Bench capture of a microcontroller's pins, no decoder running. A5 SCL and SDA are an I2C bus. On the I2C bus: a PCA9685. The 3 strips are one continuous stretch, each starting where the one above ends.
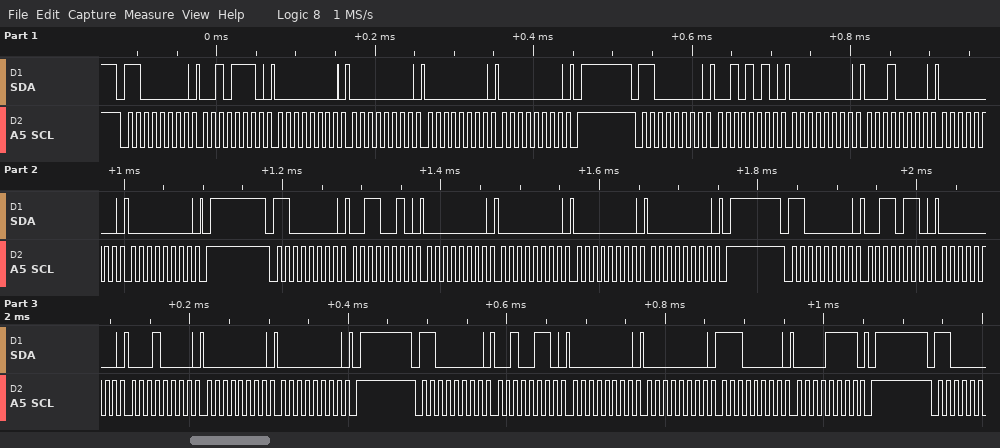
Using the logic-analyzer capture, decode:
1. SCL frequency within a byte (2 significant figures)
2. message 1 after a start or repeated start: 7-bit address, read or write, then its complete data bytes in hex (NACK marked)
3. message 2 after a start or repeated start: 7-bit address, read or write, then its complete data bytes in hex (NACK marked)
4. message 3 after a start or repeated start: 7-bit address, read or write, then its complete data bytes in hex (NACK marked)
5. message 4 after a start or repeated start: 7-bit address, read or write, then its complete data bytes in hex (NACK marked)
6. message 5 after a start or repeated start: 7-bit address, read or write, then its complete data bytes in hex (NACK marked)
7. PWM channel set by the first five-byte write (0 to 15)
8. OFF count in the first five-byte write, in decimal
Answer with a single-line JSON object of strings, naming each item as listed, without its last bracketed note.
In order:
{"SCL frequency within a byte": "100 kHz", "message 1 after a start or repeated start: 7-bit address, read or write, then its complete data bytes in hex": "0x60 write: 2E 00 00 00 00", "message 2 after a start or repeated start: 7-bit address, read or write, then its complete data bytes in hex": "0x60 write: 2A 00 10 00 00", "message 3 after a start or repeated start: 7-bit address, read or write, then its complete data bytes in hex": "0x60 write: 32 00 00 00 00", "message 4 after a start or repeated start: 7-bit address, read or write, then its complete data bytes in hex": "0x60 write: 36 00 10 00 00", "message 5 after a start or repeated start: 7-bit address, read or write, then its complete data bytes in hex": "0x60 write: 26 00 00 E0 0F", "PWM channel set by the first five-byte write": "10", "OFF count in the first five-byte write, in decimal": "0"}
